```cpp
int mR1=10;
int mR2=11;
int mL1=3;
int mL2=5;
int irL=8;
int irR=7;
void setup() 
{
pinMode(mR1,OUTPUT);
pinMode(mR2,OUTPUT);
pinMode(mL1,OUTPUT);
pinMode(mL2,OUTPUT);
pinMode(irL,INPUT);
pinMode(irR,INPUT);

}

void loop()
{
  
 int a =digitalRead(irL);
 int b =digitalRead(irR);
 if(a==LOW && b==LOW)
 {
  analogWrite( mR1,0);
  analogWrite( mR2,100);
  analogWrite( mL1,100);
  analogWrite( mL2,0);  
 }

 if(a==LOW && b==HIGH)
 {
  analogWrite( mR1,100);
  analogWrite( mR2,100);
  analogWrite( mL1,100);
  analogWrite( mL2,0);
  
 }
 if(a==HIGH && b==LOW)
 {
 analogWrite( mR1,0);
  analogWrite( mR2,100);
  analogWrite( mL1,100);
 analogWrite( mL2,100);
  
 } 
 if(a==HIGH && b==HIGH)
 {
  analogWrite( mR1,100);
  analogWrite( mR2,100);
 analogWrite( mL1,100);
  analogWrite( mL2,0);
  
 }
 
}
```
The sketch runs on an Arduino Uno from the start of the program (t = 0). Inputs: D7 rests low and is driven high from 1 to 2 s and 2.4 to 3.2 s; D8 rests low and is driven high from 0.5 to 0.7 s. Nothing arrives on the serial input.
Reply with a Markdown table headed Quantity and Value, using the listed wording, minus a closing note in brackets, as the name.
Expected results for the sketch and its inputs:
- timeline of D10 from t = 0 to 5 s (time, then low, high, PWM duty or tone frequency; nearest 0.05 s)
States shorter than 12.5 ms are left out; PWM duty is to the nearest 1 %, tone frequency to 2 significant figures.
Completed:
| Quantity | Value |
|---|---|
| timeline of D10 from t = 0 to 5 s | 0 s low; 1 s PWM 39 %; 2 s low; 2.4 s PWM 39 %; 3.2 s low |
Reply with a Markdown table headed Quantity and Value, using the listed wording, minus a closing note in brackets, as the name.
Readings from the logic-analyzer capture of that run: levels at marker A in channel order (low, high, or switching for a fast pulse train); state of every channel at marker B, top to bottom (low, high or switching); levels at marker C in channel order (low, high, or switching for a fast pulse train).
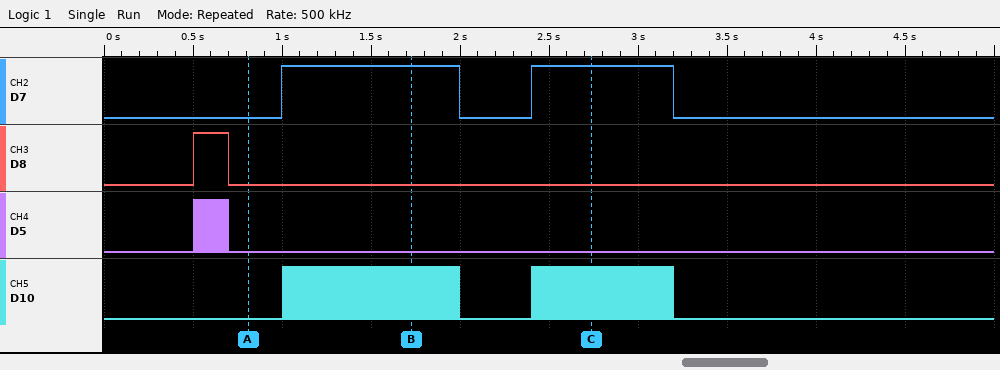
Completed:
| Quantity | Value |
|---|---|
| levels at marker A in channel order | D7 low, D8 low, D5 low, D10 low |
| state of every channel at marker B, top to bottom | D7 high, D8 low, D5 low, D10 switching |
| levels at marker C in channel order | D7 high, D8 low, D5 low, D10 switching |
